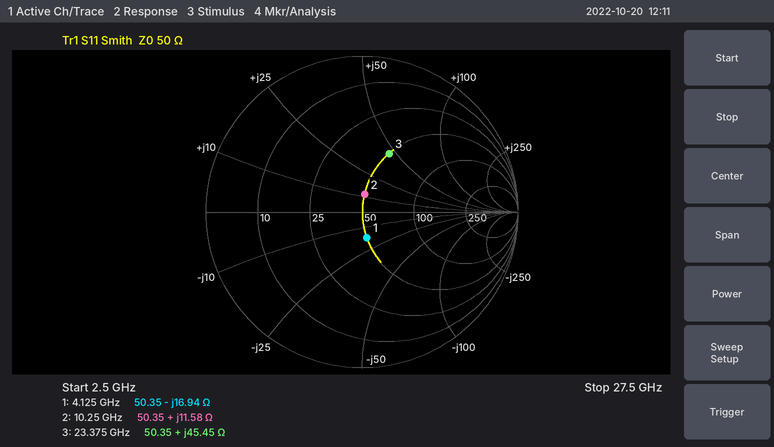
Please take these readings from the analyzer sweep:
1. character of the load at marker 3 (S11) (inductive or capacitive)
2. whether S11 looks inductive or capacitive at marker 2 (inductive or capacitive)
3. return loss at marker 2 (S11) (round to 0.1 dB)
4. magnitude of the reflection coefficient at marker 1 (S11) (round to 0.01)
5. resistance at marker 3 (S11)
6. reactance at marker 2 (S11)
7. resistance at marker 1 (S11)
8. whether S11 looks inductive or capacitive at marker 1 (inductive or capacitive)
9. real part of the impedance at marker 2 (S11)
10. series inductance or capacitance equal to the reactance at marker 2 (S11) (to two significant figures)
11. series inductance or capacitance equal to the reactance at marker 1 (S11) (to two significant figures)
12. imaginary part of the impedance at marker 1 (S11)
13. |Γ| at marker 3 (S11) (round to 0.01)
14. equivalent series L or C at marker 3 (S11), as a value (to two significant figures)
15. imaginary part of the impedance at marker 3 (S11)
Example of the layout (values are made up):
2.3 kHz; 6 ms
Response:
inductive; inductive; 18.8 dB; 0.17; 50.35 Ω; +11.58 Ω; 50.35 Ω; capacitive; 50.35 Ω; 180 pH; 2.3 pF; -16.94 Ω; 0.41; 310 pH; +45.45 Ω
